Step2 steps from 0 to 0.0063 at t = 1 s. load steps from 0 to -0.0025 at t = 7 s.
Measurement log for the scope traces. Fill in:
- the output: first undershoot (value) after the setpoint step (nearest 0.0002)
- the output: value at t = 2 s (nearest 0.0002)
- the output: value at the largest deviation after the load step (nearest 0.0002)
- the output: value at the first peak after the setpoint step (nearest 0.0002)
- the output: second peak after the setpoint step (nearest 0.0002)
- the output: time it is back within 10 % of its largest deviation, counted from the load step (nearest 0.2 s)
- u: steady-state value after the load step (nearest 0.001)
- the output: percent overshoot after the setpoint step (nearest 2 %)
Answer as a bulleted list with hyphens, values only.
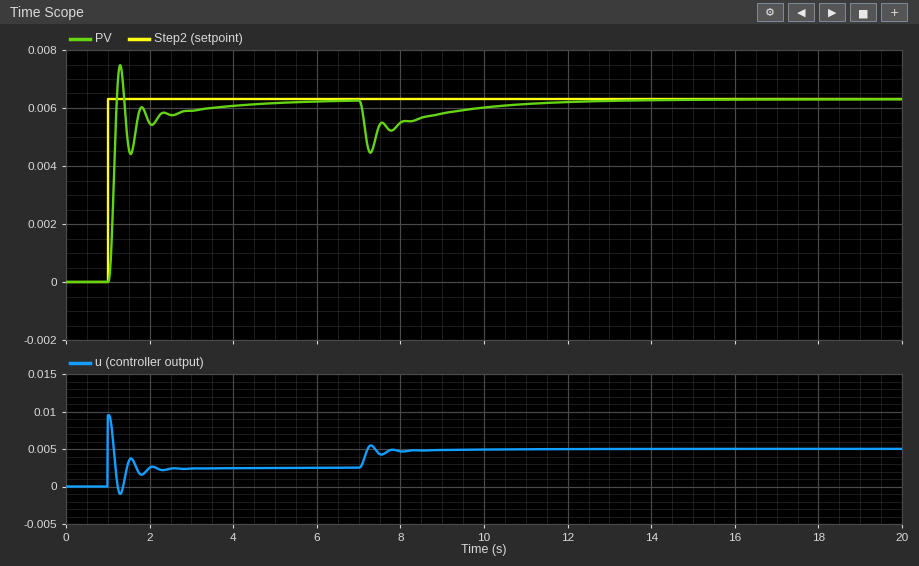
- 0.0044
- 0.0054
- 0.0044
- 0.0074
- 0.0060
- 3.8 s
- 0.005
- 18 %
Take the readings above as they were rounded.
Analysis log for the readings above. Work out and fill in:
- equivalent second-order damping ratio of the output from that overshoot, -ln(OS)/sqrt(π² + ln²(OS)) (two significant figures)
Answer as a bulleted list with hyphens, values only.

- 0.48
